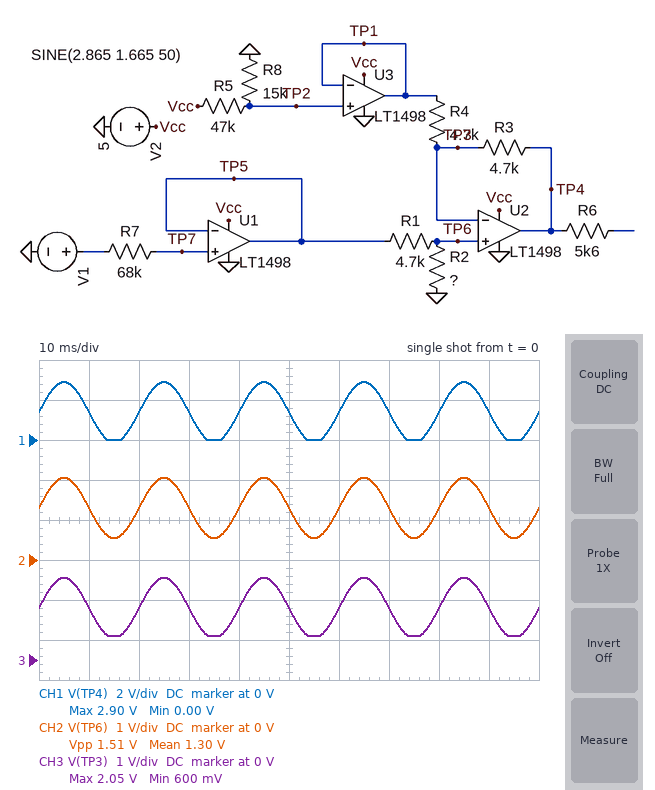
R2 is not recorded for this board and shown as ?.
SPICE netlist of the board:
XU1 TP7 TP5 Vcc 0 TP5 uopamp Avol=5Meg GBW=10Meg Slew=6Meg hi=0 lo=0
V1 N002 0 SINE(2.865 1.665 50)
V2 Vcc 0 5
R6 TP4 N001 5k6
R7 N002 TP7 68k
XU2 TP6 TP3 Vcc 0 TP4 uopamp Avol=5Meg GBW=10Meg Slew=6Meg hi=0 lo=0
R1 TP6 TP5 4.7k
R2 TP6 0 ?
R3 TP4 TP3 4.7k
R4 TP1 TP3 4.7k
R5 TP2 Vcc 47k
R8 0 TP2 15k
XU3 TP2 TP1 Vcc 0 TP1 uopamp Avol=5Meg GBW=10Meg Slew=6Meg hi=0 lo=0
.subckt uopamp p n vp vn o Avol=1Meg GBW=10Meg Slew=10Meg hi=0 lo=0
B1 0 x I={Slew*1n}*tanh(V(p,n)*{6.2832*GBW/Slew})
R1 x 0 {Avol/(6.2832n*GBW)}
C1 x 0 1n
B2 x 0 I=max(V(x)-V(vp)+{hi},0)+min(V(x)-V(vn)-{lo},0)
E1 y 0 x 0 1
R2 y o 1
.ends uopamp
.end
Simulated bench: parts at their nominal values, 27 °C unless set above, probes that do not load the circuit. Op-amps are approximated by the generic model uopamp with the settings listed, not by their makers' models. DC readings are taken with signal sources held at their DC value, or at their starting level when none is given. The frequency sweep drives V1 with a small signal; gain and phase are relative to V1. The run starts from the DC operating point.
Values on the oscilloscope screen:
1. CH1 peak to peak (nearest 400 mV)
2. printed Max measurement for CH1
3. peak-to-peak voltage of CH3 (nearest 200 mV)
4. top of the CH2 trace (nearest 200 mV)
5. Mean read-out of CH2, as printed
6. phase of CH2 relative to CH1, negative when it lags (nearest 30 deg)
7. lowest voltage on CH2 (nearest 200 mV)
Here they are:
2.8 V
2.90 V
1.4 V
2.0 V
1.30 V
0 deg
600 mV
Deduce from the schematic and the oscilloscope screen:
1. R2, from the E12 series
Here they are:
3.9 kΩ
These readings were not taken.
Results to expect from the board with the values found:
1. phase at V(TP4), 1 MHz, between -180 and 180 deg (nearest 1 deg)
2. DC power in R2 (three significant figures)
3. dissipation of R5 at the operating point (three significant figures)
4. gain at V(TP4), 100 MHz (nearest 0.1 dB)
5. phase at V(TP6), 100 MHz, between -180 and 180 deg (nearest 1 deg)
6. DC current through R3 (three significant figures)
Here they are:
-17 deg
433 µW
306 µW
-46.9 dB
-84 deg
19.1 µA
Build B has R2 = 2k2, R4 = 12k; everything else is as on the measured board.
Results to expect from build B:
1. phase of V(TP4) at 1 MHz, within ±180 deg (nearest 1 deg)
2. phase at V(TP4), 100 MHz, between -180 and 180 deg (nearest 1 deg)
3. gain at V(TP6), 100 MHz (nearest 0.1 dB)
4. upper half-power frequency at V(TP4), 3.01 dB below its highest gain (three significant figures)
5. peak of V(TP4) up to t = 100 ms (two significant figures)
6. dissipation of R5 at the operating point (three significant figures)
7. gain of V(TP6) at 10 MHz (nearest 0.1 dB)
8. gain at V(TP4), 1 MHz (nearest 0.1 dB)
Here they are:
-14 deg
-170 deg
-30.0 dB
5.35 MHz
1.5 V
306 µW
-12.9 dB
-7.2 dB
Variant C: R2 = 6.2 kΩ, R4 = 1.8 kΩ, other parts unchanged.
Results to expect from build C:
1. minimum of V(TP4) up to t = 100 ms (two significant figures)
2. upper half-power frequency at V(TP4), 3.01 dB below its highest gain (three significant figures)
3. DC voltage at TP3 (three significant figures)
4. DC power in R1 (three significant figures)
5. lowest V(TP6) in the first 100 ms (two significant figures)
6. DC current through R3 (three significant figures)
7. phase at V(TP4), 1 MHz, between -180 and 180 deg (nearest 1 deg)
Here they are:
-5.6 mV
2.59 MHz
1.63 V
325 µW
680 mV
233 µA
-26 deg
